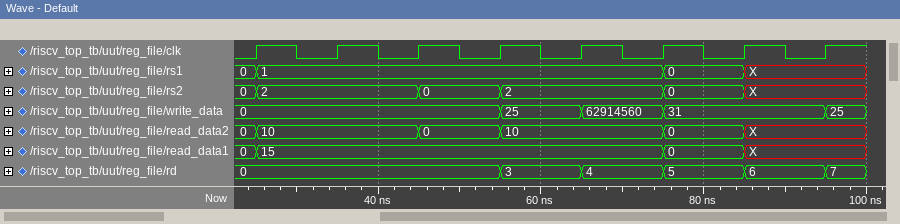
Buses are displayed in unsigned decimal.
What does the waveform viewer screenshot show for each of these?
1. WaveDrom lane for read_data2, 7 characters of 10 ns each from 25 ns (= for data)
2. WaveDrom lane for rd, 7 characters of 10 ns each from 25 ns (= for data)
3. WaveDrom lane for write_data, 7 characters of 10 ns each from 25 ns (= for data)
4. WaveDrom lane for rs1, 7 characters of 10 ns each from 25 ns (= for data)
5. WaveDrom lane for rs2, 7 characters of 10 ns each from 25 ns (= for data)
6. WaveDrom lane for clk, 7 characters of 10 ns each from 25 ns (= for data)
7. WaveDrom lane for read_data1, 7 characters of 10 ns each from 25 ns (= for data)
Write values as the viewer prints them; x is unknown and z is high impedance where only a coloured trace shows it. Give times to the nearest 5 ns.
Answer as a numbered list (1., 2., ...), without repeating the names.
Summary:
1. {name: 'read_data2', wave: '=.==.==', data: '10 0 10 0 X'}
2. {name: 'rd', wave: '=..====', data: '0 3 4 5 6'}
3. {name: 'write_data', wave: '=..===.', data: '0 25 62914560 31'}
4. {name: 'rs1', wave: '=....==', data: '1 0 X'}
5. {name: 'rs2', wave: '=.==.==', data: '2 0 2 0 X'}
6. {name: 'clk', wave: 'p......'}
7. {name: 'read_data1', wave: '=....==', data: '15 0 X'}
